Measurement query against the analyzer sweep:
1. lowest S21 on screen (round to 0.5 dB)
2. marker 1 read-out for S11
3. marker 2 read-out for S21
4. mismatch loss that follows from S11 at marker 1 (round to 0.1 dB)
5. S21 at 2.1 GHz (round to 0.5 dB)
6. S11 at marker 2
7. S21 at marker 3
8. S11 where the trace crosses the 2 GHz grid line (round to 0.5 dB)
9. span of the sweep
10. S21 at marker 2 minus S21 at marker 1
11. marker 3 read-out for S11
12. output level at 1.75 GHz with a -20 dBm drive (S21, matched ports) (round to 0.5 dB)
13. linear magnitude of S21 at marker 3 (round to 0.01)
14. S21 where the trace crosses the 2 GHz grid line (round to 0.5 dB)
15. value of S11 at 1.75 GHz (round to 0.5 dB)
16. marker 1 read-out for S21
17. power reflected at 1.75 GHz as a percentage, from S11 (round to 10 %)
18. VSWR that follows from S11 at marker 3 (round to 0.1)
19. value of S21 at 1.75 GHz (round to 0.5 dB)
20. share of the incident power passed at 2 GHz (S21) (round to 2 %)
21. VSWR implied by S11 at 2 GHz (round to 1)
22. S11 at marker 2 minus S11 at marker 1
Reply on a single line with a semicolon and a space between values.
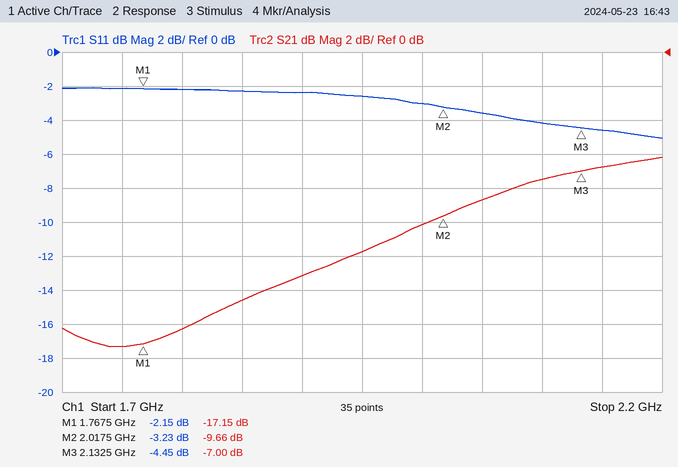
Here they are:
-17.5 dB; -2.15 dB; -9.66 dB; 4.1 dB; -7.5 dB; -3.23 dB; -7.00 dB; -3.0 dB; 500 MHz; 7.49 dB; -4.45 dB; -37.5 dBm; 0.45; -10.0 dB; -2.0 dB; -17.15 dB; 60 %; 4.0; -17.5 dB; 10 %; 6; -1.08 dB
